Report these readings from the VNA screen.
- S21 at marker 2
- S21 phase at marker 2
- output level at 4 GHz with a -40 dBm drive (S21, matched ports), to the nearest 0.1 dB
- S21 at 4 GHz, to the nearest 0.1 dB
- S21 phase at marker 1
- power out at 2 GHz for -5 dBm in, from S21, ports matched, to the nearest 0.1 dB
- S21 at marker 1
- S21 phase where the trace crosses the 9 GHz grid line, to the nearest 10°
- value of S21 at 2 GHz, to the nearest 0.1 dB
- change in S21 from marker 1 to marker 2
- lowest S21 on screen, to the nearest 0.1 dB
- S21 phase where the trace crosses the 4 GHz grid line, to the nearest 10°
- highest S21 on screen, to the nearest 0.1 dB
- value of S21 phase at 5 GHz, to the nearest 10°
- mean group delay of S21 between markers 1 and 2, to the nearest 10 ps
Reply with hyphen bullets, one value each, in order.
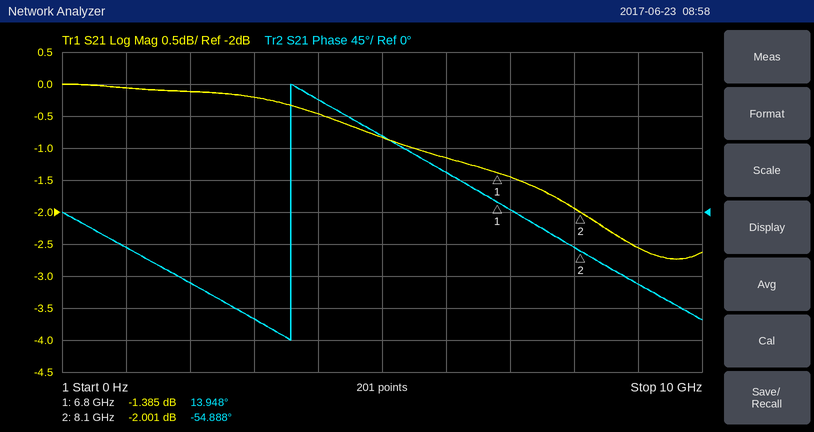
- -2.001 dB
- -54.888°
- -40.5 dBm
- -0.5 dB
- 13.948°
- -5.1 dBm
- -1.385 dB
- -100°
- -0.1 dB
- -0.616 dB
- -2.7 dB
- 160°
- 0.0 dB
- 110°
- 150 ps
